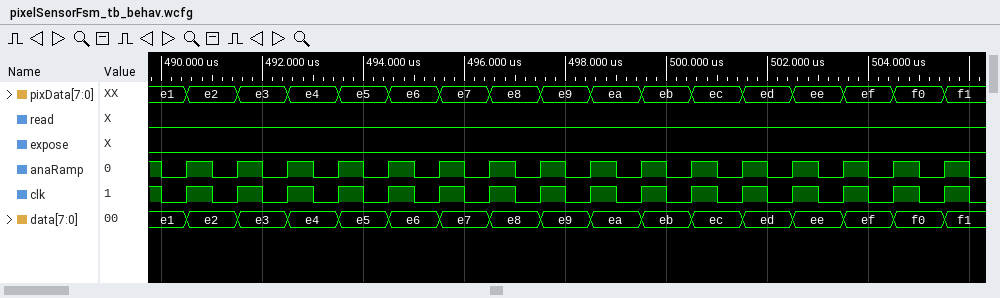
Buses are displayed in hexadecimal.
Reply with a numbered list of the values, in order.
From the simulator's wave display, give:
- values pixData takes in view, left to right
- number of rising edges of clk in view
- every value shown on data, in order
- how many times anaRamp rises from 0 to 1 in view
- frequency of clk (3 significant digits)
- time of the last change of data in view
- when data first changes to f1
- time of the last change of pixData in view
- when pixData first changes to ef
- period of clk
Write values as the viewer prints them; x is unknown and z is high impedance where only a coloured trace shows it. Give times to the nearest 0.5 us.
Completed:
1. e1, e2, e3, e4, e5, e6, e7, e8, e9, ea, eb, ec, ed, ee, ef, f0, f1
2. 16
3. e1, e2, e3, e4, e5, e6, e7, e8, e9, ea, eb, ec, ed, ee, ef, f0, f1
4. 16
5. 1.00 MHz
6. 505.5 us
7. 505.5 us
8. 505.5 us
9. 503.5 us
10. 1 us
